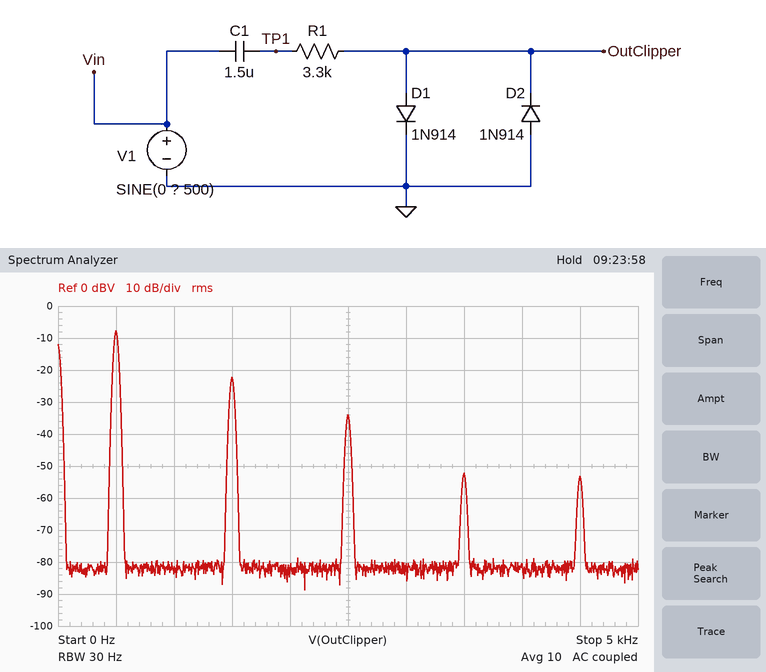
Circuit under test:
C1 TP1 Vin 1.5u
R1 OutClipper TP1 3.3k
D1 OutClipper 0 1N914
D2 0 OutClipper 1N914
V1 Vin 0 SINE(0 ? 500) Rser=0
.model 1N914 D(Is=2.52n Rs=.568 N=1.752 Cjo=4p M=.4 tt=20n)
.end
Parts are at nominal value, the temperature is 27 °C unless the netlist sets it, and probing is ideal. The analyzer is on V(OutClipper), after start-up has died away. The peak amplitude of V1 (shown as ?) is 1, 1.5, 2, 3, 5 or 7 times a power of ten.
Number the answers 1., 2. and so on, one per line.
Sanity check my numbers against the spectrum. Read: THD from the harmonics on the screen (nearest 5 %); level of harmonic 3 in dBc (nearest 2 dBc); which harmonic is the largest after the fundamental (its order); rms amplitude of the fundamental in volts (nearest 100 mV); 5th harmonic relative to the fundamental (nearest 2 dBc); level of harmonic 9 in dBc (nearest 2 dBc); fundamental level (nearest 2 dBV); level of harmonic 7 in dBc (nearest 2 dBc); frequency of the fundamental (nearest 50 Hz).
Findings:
1. 20 %
2. -14 dBc
3. 3
4. 400 mV
5. -26 dBc
6. -46 dBc
7. -8 dBV
8. -44 dBc
9. 500 Hz
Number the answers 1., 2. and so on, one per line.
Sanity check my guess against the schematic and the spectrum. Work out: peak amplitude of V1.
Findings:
1. 1 V
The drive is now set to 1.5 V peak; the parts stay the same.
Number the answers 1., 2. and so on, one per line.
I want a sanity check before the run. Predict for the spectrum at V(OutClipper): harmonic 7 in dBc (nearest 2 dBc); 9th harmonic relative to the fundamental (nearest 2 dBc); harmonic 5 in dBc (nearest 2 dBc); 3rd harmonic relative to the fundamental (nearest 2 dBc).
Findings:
1. -28 dBc
2. -38 dBc
3. -20 dBc
4. -12 dBc
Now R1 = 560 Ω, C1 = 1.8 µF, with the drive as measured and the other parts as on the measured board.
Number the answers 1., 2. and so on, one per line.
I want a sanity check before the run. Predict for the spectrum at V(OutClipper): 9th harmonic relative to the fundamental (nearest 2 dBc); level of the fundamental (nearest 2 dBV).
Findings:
1. -42 dBc
2. -6 dBV
